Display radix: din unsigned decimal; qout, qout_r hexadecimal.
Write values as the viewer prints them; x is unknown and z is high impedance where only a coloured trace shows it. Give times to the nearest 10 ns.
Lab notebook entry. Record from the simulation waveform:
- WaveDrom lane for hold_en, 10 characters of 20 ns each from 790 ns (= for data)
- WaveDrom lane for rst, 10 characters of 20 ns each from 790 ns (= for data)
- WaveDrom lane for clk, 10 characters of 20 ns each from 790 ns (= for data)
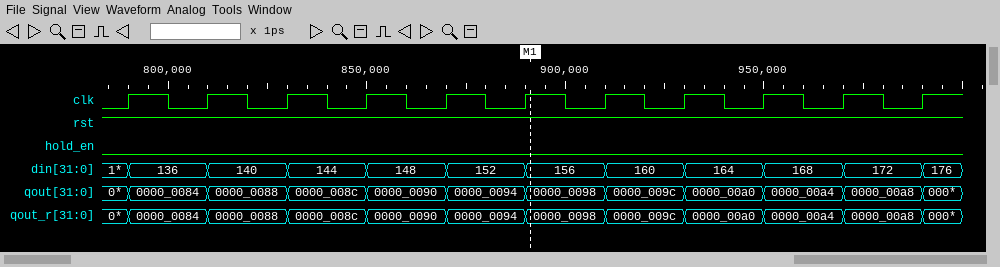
{name: 'hold_en', wave: '0.........'}
{name: 'rst', wave: '1.........'}
{name: 'clk', wave: 'p.........'}
